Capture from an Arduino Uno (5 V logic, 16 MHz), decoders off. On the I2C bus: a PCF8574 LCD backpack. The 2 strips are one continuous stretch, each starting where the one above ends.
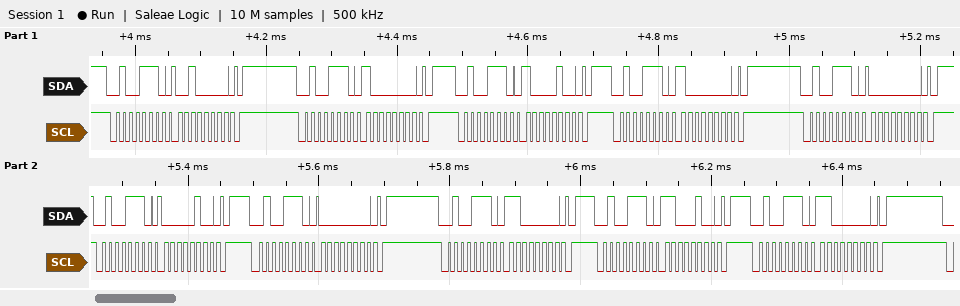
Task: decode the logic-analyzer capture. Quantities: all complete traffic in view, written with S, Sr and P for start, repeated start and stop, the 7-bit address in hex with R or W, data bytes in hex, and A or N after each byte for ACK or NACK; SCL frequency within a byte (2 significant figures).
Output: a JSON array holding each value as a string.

["S 27W A 20 A P S 27W A 80 A P S 27W A 84 A P S 27W A 80 A P S 27W A 00 A P S 27W A 04 A P S 27W A 00 A P S 27W A C0 A P S 27W A C4 A P S 27W A C0 A P", "100 kHz"]
